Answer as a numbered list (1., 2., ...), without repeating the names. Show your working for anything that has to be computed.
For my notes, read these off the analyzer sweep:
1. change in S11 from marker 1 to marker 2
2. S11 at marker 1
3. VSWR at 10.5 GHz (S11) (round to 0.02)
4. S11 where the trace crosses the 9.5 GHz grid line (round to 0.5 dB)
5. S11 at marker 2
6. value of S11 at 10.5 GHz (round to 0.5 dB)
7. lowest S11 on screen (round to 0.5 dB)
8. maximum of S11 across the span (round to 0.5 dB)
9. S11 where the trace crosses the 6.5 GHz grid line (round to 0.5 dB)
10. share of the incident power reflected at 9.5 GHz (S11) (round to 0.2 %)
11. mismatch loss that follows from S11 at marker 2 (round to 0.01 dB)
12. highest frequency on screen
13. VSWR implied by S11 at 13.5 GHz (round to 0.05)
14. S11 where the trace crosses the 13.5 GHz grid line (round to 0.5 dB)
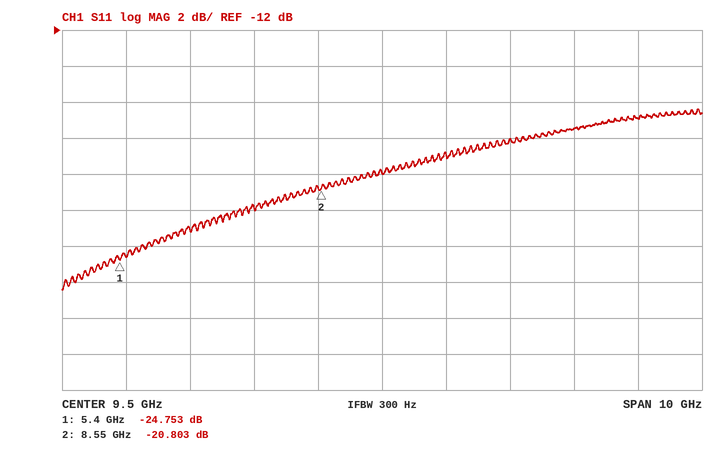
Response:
1. -20.803 − (-24.753) = 3.950 dB
2. -24.753 dB
3. |Γ| = 10^(-19/20) = 0.1122; VSWR = (1 + 0.1122)/(1 − 0.1122) ≈ 1.25, so 1.26 to the nearest 0.02
4. -20.0 dB
5. -20.803 dB
6. -19.0 dB
7. -26.5 dB
8. -16.5 dB
9. -23.0 dB
10. 10^(-20/10) ≈ 1.0 %
11. −10 log10(1 − 10^(-20.803/10)) ≈ 0.04 dB
12. 14.5 GHz
13. |Γ| = 10^(-17/20) = 0.1413; VSWR = (1 + 0.1413)/(1 − 0.1413) ≈ 1.33, so 1.35 to the nearest 0.05
14. -17.0 dB
